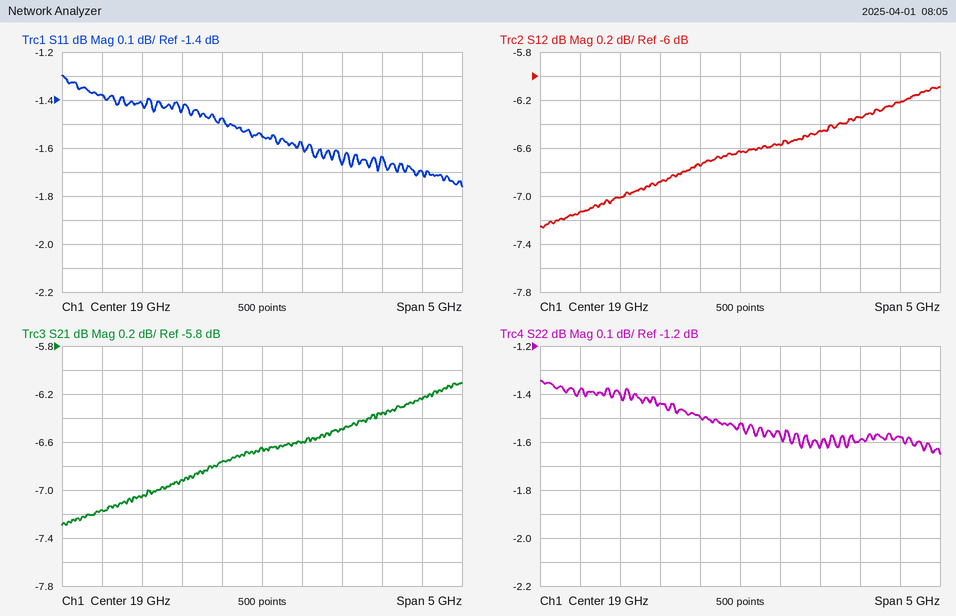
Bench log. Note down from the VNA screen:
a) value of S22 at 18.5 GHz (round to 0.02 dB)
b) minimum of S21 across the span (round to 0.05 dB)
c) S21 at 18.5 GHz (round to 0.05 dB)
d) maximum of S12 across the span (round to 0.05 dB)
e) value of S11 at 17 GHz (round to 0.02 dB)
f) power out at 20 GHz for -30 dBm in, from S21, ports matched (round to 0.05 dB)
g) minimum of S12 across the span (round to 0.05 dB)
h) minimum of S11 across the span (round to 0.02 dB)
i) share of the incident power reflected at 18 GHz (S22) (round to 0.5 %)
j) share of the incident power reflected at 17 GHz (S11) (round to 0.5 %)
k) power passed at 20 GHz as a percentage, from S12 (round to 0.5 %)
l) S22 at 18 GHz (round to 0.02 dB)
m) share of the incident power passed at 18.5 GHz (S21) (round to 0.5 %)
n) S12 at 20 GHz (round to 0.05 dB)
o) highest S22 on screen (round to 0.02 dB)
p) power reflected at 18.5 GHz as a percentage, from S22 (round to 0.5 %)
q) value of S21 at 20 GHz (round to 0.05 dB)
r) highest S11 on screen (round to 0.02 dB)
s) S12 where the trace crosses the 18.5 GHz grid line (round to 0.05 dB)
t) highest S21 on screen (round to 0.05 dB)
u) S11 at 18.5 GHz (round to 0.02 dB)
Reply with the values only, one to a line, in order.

-1.50 dB
-7.30 dB
-6.75 dB
-6.10 dB
-1.38 dB
-36.50 dBm
-7.25 dB
-1.76 dB
72.0 %
73.0 %
22.5 %
-1.44 dB
21.0 %
-6.45 dB
-1.34 dB
71.0 %
-6.50 dB
-1.30 dB
-6.75 dB
-6.10 dB
-1.48 dB
